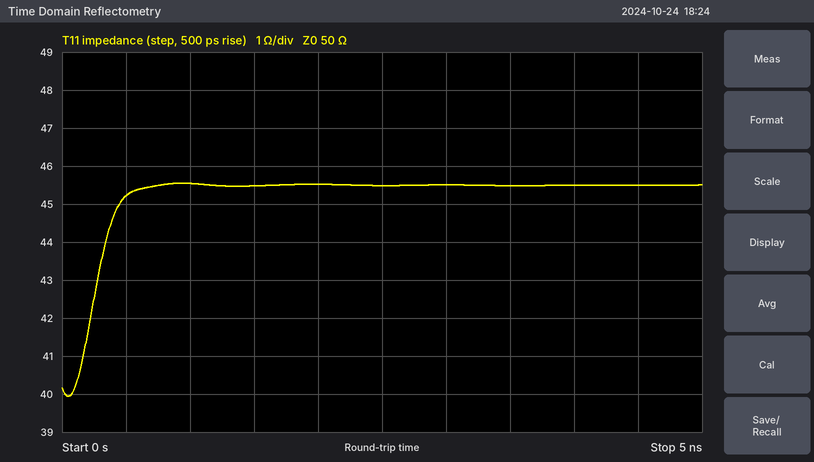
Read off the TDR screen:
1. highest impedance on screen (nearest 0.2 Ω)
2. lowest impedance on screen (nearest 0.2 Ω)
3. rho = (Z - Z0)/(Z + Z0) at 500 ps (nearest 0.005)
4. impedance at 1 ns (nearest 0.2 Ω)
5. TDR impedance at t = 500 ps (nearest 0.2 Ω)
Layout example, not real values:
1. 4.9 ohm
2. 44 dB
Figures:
1. 45.6 Ω
2. 40.0 Ω
3. -0.050
4. 45.6 Ω
5. 45.2 Ω
